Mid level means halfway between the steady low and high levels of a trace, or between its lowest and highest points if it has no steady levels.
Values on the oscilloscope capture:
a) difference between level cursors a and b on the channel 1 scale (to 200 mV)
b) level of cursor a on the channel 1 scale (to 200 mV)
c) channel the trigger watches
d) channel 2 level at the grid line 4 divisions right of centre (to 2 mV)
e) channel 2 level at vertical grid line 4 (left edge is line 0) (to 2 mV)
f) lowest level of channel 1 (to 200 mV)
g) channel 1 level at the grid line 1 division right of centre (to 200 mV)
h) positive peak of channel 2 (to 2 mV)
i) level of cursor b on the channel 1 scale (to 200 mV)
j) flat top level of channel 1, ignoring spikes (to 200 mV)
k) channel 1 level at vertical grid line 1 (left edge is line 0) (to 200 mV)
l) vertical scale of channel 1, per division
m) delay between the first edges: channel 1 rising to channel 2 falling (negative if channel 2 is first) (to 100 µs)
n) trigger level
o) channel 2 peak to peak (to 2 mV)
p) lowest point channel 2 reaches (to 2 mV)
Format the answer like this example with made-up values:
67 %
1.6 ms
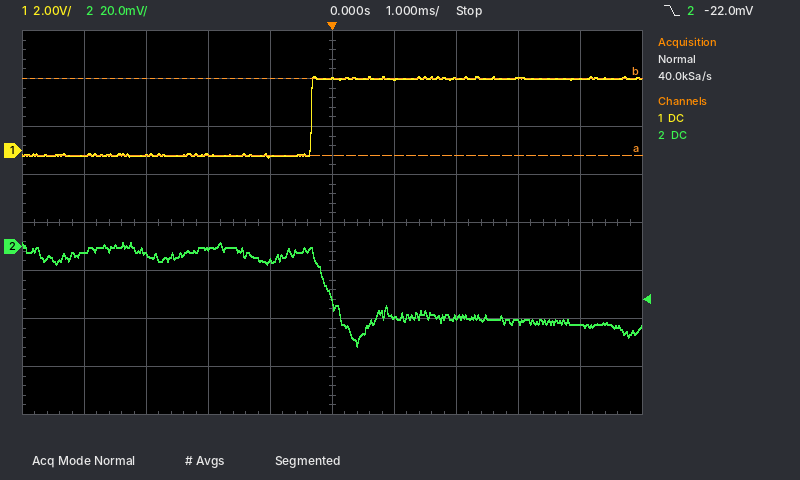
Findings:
3.2 V
-200 mV
channel 2
-32 mV
-6 mV
-200 mV
3.0 V
2 mV
3.0 V
3.0 V
-200 mV
2 V
+300 µs
-22.0 mV
44 mV
-42 mV
